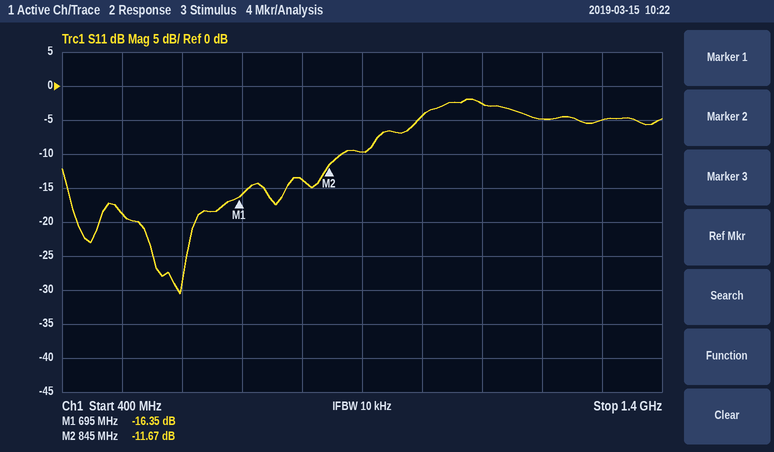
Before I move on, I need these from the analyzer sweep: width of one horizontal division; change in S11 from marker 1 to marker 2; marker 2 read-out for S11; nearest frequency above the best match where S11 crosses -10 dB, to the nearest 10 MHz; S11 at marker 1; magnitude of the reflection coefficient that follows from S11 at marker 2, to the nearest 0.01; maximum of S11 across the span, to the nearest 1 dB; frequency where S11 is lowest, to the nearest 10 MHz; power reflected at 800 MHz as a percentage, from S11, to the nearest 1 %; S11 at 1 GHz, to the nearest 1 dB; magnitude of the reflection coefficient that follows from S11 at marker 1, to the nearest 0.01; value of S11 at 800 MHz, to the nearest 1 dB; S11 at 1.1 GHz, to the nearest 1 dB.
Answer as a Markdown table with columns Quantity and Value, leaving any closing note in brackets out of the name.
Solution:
| Quantity | Value |
|---|---|
| width of one horizontal division | 100 MHz |
| change in S11 from marker 1 to marker 2 | 4.68 dB |
| marker 2 read-out for S11 | -11.67 dB |
| nearest frequency above the best match where S11 crosses -10 dB, to the nearest 10 MHz | 870 MHz |
| S11 at marker 1 | -16.35 dB |
| magnitude of the reflection coefficient that follows from S11 at marker 2, to the nearest 0.01 | 0.26 |
| maximum of S11 across the span, to the nearest 1 dB | -2 dB |
| frequency where S11 is lowest, to the nearest 10 MHz | 600 MHz |
| power reflected at 800 MHz as a percentage, from S11, to the nearest 1 % | 4 % |
| S11 at 1 GHz, to the nearest 1 dB | -4 dB |
| magnitude of the reflection coefficient that follows from S11 at marker 1, to the nearest 0.01 | 0.15 |
| value of S11 at 800 MHz, to the nearest 1 dB | -14 dB |
| S11 at 1.1 GHz, to the nearest 1 dB | -3 dB |
